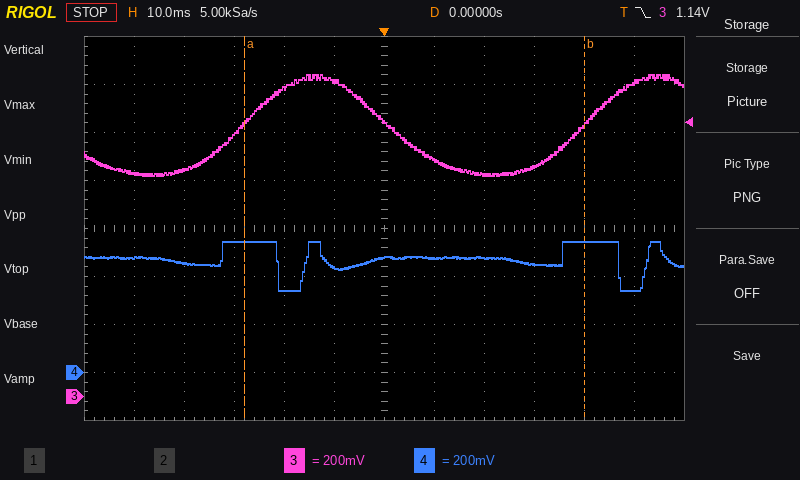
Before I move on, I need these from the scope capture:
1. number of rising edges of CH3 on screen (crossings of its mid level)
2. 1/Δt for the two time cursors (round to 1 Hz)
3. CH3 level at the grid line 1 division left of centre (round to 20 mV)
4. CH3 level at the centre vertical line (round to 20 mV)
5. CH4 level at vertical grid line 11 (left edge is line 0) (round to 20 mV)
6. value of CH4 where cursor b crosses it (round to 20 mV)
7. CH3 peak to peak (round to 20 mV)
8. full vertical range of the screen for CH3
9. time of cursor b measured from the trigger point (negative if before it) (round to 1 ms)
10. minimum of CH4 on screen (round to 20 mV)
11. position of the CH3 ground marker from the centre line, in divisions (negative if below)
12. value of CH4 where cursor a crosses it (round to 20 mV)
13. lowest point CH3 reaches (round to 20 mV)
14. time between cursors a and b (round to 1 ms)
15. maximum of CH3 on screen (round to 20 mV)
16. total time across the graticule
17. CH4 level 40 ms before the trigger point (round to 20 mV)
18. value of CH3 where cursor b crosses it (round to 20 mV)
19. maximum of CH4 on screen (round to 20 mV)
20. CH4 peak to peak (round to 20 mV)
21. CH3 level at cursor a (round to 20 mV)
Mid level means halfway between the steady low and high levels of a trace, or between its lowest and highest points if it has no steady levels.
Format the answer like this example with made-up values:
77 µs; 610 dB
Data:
2; 15 Hz; 1.32 V; 1.14 V; 340 mV; 540 mV; 420 mV; 1.6 V; +40 ms; 340 mV; -3.5 div; 540 mV; 920 mV; 68 ms; 1.34 V; 120 ms; 460 mV; 1.14 V; 540 mV; 200 mV; 1.14 V
